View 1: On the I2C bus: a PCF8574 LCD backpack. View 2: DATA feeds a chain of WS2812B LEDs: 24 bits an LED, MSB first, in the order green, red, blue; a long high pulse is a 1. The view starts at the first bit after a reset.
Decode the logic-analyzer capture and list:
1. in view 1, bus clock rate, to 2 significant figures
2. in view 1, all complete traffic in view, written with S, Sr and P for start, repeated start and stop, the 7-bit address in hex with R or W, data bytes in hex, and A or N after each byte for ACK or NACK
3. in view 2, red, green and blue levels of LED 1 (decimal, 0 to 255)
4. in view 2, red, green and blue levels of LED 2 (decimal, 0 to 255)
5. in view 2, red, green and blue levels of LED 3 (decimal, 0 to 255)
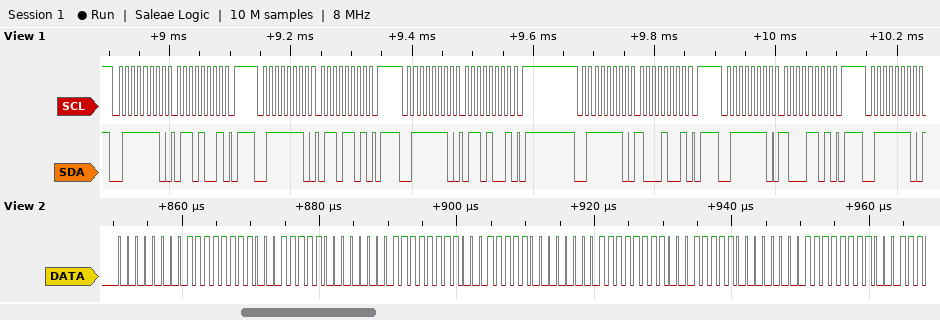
100 kHz
S 3FW A 69 A P S 3FW A 6D A P S 3FW A 69 A P S 3FW A 89 A P S 3FW A 8D A P S 3FW A
255, 0, 31
255, 0, 31
255, 0, 31
